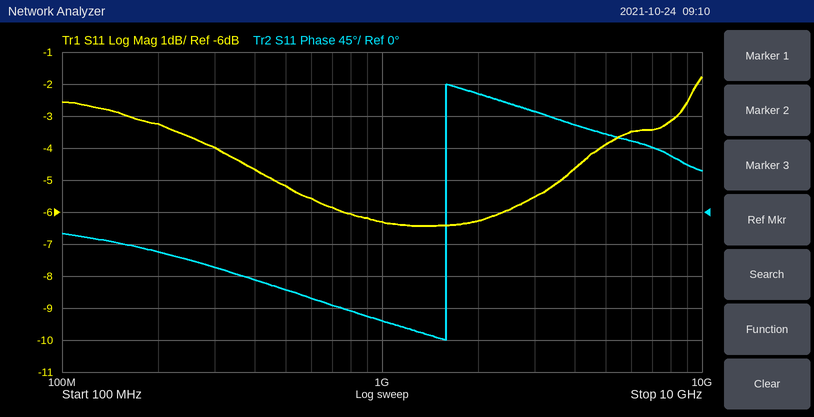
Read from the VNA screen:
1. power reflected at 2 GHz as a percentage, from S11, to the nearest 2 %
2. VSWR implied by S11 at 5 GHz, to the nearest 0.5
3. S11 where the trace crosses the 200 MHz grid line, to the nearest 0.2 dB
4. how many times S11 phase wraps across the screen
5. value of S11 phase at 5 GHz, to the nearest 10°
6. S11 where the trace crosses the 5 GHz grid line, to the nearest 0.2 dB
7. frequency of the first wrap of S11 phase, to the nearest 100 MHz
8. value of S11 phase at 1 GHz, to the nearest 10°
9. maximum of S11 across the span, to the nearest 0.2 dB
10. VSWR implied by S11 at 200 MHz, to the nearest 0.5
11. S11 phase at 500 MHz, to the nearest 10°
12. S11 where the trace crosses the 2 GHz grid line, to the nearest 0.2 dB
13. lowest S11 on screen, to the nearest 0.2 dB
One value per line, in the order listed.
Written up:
24 %
4.5
-3.2 dB
1
110°
-3.8 dB
1.6 GHz
-150°
-1.8 dB
5.5
-110°
-6.2 dB
-6.4 dB
